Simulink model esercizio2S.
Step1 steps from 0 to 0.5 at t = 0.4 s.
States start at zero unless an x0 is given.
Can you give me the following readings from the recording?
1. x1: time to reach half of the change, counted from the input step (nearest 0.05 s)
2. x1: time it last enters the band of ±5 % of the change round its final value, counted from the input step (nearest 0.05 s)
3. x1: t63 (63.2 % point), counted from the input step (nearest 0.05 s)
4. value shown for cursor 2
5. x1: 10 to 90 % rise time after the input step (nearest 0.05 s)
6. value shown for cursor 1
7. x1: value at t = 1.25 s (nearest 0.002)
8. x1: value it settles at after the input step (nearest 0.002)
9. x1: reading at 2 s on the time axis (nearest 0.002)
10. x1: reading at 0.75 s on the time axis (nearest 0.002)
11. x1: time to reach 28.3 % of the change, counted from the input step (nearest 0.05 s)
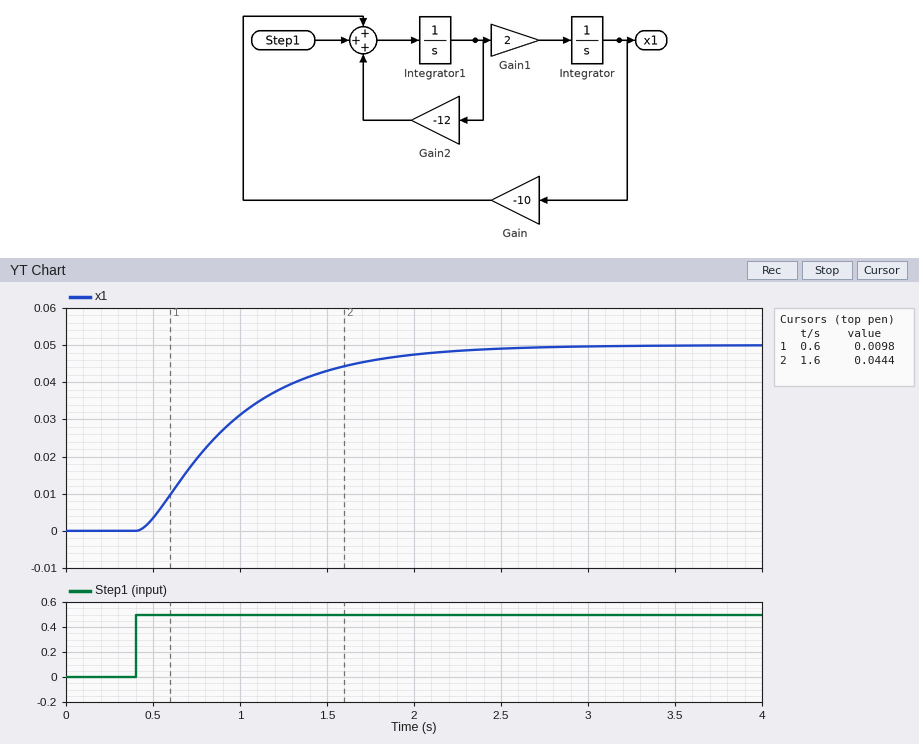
0.45 s
1.60 s
0.60 s
0.0444
1.15 s
0.0098
0.038
0.050
0.048
0.020
0.25 s
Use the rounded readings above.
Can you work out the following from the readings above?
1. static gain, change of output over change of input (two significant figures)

0.10
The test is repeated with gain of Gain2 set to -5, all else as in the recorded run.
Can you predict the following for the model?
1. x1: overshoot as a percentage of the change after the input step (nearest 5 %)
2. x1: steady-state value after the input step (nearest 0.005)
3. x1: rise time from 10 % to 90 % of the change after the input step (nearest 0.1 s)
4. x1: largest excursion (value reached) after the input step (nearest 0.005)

10 %
0.050
0.4 s
0.055
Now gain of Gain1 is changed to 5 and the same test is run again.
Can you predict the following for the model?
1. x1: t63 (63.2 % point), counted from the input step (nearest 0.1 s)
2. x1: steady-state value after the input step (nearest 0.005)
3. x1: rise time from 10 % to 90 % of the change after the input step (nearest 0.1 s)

0.3 s
0.050
0.4 s
